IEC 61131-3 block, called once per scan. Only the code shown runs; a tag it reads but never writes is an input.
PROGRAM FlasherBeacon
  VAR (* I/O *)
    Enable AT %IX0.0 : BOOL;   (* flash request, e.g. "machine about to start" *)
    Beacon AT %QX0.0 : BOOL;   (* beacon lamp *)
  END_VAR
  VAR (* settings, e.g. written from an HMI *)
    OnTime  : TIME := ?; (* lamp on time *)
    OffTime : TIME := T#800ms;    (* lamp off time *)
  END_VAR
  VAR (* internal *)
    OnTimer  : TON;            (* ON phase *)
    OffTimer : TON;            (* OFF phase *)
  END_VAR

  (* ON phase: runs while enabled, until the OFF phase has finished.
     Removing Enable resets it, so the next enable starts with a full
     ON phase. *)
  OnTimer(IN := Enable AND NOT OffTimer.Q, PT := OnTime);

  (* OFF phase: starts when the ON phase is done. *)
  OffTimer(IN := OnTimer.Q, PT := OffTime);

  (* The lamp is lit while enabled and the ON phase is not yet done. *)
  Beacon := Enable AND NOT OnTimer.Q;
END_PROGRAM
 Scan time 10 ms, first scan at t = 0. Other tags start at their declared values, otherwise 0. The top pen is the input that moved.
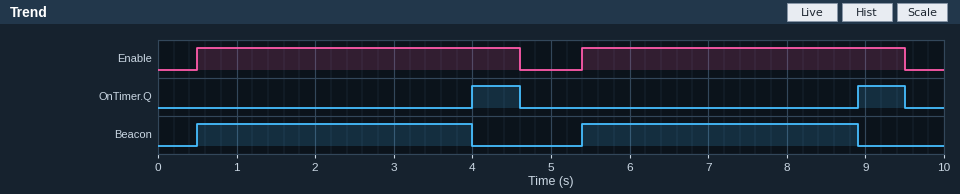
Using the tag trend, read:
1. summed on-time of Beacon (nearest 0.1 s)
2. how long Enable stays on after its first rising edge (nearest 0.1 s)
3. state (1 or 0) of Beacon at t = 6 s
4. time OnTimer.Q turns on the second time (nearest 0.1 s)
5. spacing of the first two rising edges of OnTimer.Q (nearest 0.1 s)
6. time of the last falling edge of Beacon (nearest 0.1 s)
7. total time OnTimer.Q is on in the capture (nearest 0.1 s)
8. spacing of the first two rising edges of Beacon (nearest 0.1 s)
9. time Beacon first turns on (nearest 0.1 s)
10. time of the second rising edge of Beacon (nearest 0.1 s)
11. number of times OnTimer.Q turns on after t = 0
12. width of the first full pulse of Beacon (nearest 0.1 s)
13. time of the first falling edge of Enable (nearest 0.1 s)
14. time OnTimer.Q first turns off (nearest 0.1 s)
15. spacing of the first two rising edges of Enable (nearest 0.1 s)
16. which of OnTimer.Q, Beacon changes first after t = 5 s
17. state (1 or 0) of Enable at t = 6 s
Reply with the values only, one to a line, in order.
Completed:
7.0 s
4.1 s
1
8.9 s
4.9 s
8.9 s
1.2 s
4.9 s
0.5 s
5.4 s
2
3.5 s
4.6 s
4.6 s
4.9 s
Beacon
1
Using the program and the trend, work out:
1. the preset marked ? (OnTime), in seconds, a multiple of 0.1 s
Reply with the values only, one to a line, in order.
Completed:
3.5 s
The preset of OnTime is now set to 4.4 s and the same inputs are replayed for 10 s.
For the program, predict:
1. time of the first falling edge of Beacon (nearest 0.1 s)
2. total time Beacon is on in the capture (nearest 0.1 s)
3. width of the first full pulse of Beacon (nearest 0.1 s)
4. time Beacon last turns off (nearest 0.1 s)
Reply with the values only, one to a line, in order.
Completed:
4.6 s
8.2 s
4.1 s
9.5 s
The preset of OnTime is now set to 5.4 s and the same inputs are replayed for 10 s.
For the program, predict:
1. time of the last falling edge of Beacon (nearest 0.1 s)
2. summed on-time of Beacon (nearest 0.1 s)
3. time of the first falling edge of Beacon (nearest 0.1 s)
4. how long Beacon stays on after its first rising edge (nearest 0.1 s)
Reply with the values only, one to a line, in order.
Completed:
9.5 s
8.2 s
4.6 s
4.1 s
